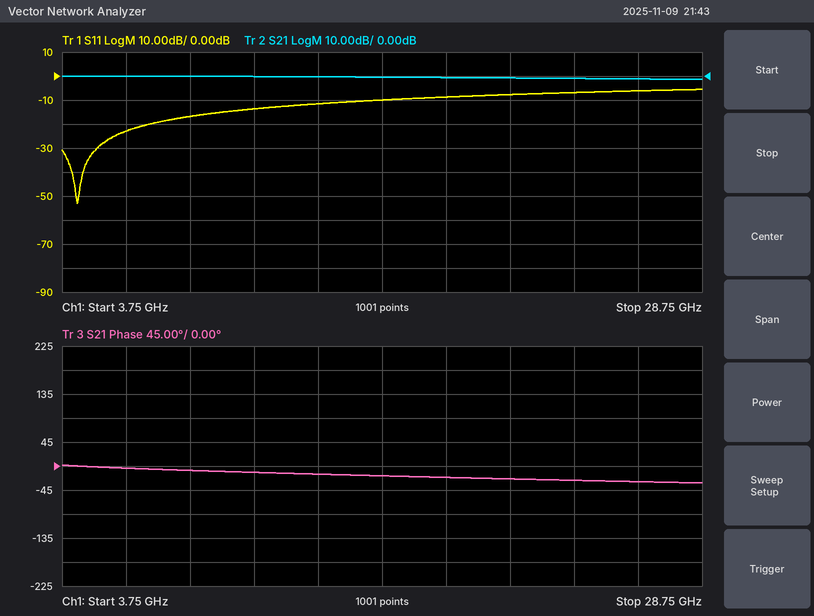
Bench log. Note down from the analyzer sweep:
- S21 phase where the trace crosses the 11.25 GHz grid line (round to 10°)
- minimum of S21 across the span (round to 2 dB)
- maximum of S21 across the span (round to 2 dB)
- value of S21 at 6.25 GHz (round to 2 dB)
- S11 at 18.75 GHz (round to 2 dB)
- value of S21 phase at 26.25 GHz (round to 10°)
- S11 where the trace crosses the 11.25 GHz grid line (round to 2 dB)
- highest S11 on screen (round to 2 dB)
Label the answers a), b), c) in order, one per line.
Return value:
a) -10°
b) -2 dB
c) 0 dB
d) 0 dB
e) -8 dB
f) -30°
g) -14 dB
h) -6 dB
